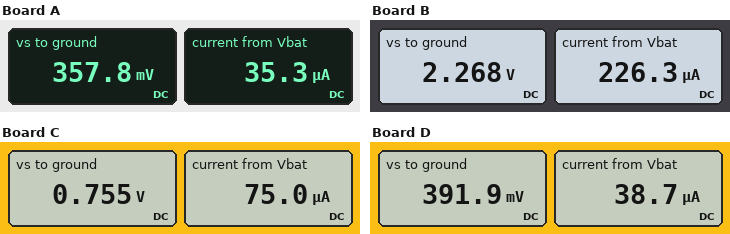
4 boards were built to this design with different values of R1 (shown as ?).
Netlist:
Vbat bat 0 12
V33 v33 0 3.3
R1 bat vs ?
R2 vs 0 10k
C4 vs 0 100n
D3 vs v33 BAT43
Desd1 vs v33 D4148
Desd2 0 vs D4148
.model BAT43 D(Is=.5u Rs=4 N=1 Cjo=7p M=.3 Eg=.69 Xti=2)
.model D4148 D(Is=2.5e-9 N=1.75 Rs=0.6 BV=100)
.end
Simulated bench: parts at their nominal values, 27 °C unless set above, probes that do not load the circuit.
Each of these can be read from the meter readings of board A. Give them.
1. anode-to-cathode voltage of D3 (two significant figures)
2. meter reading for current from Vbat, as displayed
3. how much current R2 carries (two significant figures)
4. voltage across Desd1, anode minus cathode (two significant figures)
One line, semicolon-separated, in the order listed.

-2.9 V; 35.3 µA; 36 µA; -2.9 V
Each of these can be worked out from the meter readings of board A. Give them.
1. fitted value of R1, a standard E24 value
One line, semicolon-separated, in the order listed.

330 kΩ
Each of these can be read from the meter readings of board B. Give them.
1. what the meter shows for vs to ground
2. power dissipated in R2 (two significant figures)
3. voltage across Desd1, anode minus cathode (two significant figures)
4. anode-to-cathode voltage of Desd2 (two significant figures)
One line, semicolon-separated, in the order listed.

2.268 V; 510 µW; -1.0 V; -2.3 V
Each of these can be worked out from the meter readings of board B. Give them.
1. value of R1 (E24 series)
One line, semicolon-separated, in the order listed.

43 kΩ
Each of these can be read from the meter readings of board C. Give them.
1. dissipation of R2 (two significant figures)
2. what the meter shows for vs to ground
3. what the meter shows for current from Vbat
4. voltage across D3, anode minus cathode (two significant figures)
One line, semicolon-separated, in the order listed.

57 µW; 0.755 V; 75.0 µA; -2.5 V
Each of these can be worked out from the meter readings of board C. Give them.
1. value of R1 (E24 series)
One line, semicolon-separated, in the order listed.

150 kΩ
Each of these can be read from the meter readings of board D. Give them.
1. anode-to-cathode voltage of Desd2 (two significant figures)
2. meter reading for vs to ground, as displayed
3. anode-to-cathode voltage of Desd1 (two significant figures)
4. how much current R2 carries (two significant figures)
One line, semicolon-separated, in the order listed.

-390 mV; 391.9 mV; -2.9 V; 39 µA
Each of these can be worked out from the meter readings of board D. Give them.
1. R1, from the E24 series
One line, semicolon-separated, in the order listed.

300 kΩ
